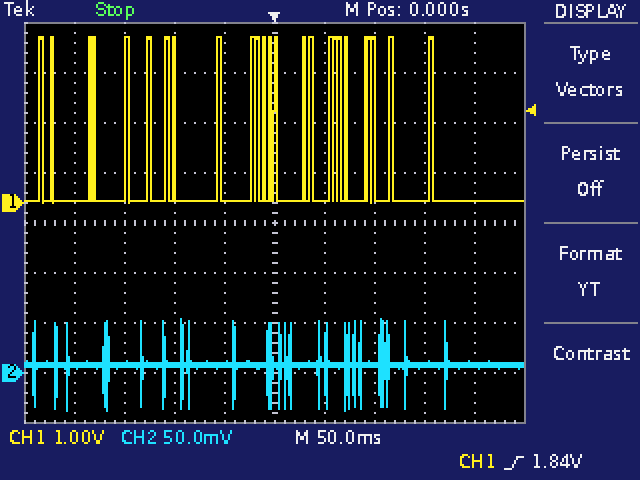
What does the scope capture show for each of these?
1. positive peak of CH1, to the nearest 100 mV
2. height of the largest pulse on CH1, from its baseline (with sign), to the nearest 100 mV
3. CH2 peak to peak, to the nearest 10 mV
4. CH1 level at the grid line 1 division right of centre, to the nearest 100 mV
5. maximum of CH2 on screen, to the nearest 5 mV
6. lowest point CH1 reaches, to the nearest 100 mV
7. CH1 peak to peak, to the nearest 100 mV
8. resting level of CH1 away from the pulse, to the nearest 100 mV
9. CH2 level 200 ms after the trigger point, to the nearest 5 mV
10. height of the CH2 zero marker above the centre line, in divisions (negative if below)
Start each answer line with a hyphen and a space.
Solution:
- 3.3 V
- +3.3 V
- 90 mV
- 0.0 V
- 55 mV
- 0.0 V
- 3.3 V
- 0.0 V
- 10 mV
- -3.0 div
